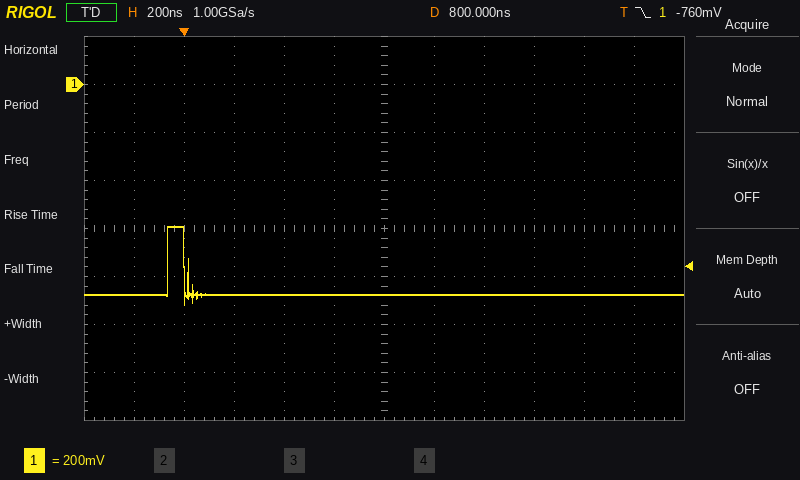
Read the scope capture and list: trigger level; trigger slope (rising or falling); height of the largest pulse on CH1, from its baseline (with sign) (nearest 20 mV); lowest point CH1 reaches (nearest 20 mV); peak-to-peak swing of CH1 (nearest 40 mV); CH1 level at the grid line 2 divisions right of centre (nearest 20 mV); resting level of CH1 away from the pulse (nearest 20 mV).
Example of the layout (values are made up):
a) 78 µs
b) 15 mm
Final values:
a) -760 mV
b) falling
c) +280 mV
d) -920 mV
e) 320 mV
f) -880 mV
g) -880 mV
